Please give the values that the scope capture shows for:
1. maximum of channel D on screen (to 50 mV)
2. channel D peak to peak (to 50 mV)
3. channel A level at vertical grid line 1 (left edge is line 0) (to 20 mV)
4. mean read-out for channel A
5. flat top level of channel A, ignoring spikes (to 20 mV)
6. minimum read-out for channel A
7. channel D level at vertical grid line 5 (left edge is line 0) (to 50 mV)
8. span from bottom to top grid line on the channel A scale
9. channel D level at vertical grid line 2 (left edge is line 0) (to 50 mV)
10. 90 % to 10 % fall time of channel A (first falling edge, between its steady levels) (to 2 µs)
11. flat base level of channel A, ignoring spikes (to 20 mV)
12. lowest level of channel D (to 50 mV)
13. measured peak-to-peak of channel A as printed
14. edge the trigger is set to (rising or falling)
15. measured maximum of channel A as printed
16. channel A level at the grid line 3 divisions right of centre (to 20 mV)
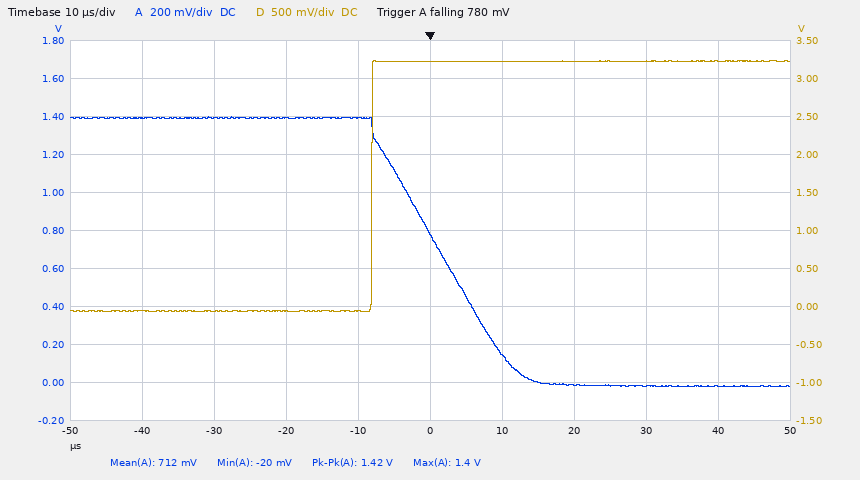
3.25 V
3.30 V
1.40 V
712 mV
1.40 V
-20 mV
3.20 V
2 V
-50 mV
18 µs
-20 mV
-50 mV
1.42 V
falling
1.4 V
-20 mV
